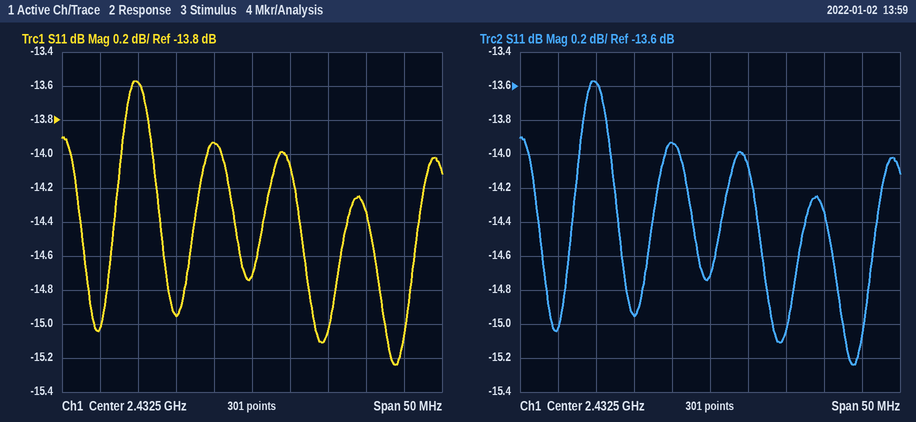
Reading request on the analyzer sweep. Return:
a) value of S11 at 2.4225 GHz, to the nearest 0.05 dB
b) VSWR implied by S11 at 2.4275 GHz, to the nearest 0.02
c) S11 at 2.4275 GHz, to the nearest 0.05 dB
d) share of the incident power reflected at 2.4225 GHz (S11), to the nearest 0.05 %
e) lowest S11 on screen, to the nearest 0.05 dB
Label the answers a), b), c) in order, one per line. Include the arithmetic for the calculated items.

a) -14.95 dB
b) |Γ| = 10^(-13.95/20) = 0.2007; VSWR = (1 + 0.2007)/(1 − 0.2007) ≈ 1.50
c) -13.95 dB
d) 10^(-14.95/10) ≈ 3.20 %
e) -15.25 dB
